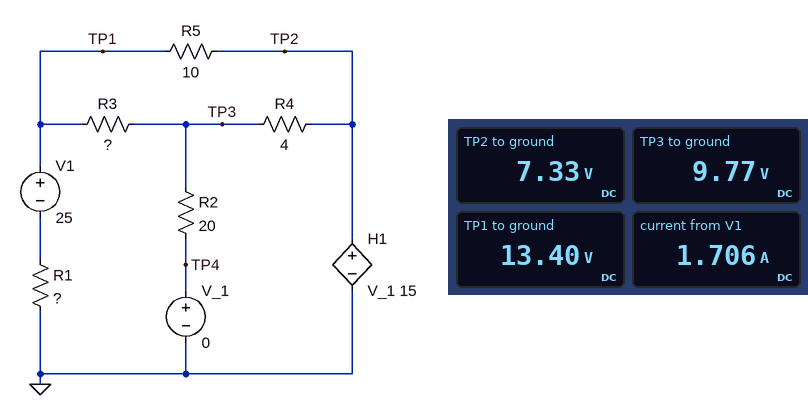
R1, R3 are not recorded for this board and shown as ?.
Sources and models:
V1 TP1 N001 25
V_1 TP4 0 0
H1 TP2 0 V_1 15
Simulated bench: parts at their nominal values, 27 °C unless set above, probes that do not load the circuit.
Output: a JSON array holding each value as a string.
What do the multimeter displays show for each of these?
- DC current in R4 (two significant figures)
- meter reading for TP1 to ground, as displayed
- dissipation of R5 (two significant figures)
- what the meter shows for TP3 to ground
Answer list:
["610 mA", "13.40 V", "3.7 W", "9.77 V"]
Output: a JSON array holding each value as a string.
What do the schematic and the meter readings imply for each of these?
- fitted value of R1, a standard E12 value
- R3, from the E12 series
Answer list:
["6.8 Ω", "3.3 Ω"]
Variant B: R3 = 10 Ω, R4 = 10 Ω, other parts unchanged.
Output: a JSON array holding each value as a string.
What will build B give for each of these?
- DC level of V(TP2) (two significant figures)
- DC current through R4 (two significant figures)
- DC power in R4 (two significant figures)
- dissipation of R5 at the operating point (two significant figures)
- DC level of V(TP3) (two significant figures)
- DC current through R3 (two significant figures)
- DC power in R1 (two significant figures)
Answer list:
["6.4 V", "210 mA", "450 mW", "7.2 W", "8.5 V", "640 mA", "15 W"]
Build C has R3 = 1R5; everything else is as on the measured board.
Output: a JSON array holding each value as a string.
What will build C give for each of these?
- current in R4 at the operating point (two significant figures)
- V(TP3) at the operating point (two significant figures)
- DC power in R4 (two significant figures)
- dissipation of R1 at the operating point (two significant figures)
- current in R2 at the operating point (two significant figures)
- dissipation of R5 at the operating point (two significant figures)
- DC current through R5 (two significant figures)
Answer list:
["700 mA", "11 V", "2.0 W", "21 W", "560 mA", "2.2 W", "470 mA"]
